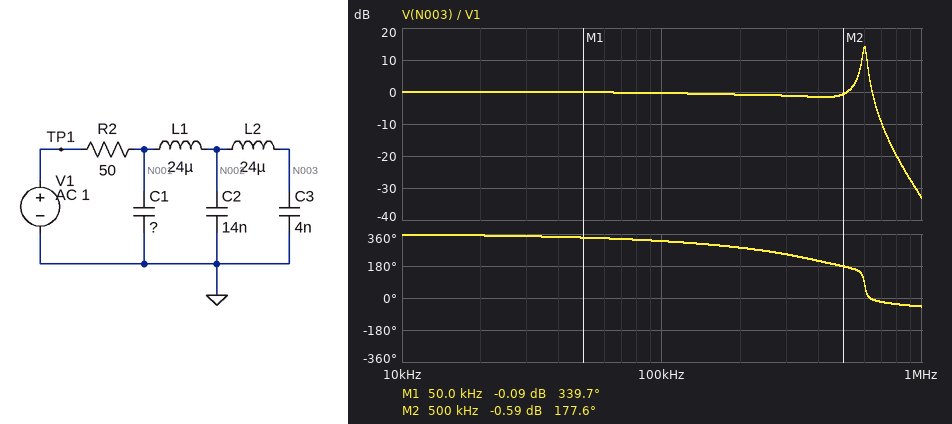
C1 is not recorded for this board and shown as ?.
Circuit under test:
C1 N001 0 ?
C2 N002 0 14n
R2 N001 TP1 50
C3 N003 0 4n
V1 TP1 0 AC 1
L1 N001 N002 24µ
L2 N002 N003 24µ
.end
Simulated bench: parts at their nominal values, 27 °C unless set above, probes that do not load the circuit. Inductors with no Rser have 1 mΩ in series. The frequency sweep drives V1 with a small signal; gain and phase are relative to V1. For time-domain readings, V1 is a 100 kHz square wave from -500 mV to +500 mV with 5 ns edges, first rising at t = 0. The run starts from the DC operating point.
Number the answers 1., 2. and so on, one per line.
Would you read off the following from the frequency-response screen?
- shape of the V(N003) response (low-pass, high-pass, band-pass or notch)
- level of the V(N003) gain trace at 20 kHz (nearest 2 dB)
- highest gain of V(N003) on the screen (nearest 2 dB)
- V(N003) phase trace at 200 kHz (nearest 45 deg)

1. low-pass
2. 0 dB
3. 14 dB
4. 270 deg
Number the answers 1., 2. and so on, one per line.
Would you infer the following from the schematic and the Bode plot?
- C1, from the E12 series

1. 4.7 nF
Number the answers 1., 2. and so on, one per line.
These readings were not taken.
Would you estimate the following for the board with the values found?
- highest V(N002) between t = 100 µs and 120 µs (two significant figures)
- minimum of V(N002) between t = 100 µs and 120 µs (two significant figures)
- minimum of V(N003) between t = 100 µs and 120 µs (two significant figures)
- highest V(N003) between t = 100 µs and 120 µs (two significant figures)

1. 520 mV
2. -520 mV
3. -580 mV
4. 580 mV
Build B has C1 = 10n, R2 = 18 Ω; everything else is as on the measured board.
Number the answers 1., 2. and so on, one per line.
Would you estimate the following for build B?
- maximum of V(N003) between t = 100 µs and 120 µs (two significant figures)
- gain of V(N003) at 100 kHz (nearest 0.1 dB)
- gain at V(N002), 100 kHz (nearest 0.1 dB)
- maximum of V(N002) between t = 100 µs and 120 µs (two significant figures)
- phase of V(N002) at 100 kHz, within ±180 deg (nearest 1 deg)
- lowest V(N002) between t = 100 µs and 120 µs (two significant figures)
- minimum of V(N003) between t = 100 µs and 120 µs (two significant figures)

1. 1.0 V
2. 1.4 dB
3. 1.1 dB
4. 910 mV
5. -20 deg
6. -910 mV
7. -1.0 V
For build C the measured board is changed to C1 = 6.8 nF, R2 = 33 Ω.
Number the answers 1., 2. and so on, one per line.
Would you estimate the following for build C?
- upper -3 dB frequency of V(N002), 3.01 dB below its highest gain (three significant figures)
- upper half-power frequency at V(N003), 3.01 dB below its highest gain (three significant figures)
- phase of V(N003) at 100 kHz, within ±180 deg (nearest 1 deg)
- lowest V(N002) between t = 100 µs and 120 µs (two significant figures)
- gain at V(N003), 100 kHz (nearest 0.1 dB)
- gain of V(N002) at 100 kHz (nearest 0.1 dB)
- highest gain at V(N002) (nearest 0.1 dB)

1. 609 kHz
2. 608 kHz
3. -31 deg
4. -690 mV
5. 0.7 dB
6. 0.3 dB
7. 9.7 dB
